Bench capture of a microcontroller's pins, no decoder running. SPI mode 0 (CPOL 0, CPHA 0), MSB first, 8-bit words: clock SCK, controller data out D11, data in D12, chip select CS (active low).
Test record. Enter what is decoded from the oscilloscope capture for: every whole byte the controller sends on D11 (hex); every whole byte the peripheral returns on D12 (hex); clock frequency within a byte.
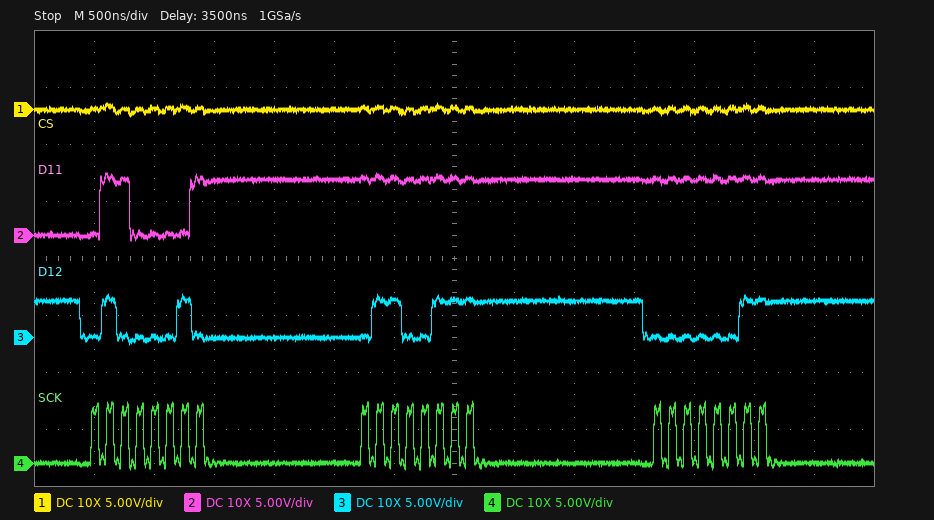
0x61 0xFF 0xFF
0x42 0x67 0x03
8 MHz
